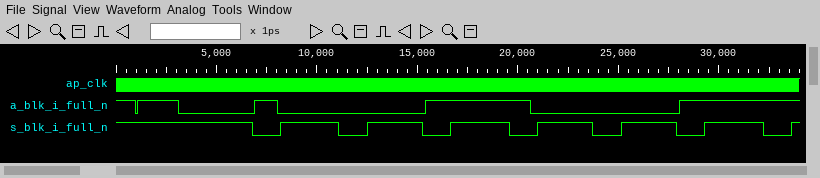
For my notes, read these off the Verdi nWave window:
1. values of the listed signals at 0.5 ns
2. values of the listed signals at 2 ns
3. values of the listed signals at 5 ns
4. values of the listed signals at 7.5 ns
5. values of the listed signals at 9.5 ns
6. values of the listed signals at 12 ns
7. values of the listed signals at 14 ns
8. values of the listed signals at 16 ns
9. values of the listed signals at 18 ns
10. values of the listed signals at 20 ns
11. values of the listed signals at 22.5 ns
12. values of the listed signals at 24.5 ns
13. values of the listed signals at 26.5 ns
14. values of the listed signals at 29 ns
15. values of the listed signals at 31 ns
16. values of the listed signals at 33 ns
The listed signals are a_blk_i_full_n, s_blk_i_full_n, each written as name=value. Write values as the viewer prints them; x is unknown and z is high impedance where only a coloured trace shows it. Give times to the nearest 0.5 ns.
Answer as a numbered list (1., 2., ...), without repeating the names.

1. a_blk_i_full_n=1, s_blk_i_full_n=1
2. a_blk_i_full_n=1, s_blk_i_full_n=1
3. a_blk_i_full_n=0, s_blk_i_full_n=1
4. a_blk_i_full_n=1, s_blk_i_full_n=0
5. a_blk_i_full_n=0, s_blk_i_full_n=1
6. a_blk_i_full_n=0, s_blk_i_full_n=0
7. a_blk_i_full_n=0, s_blk_i_full_n=1
8. a_blk_i_full_n=1, s_blk_i_full_n=0
9. a_blk_i_full_n=1, s_blk_i_full_n=1
10. a_blk_i_full_n=1, s_blk_i_full_n=0
11. a_blk_i_full_n=0, s_blk_i_full_n=1
12. a_blk_i_full_n=0, s_blk_i_full_n=0
13. a_blk_i_full_n=0, s_blk_i_full_n=1
14. a_blk_i_full_n=1, s_blk_i_full_n=0
15. a_blk_i_full_n=1, s_blk_i_full_n=1
16. a_blk_i_full_n=1, s_blk_i_full_n=0
